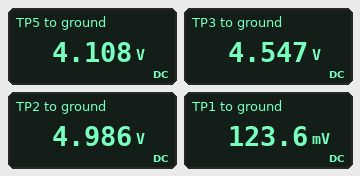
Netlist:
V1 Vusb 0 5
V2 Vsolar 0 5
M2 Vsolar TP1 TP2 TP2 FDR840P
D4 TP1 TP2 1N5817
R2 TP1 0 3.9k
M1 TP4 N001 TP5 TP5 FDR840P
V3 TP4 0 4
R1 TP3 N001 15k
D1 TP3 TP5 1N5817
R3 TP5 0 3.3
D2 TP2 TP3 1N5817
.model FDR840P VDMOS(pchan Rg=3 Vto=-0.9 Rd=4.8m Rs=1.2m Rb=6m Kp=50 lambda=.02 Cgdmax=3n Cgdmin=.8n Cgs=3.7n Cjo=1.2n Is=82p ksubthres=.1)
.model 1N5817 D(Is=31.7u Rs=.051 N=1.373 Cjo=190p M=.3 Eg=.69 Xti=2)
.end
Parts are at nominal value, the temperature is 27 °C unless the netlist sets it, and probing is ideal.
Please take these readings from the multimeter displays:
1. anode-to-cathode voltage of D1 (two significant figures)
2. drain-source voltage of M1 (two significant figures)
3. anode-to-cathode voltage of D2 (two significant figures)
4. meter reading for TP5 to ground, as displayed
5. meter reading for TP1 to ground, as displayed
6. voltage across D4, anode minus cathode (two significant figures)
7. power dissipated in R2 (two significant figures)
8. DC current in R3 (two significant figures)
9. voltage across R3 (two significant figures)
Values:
440 mV
-110 mV
440 mV
4.108 V
123.6 mV
-4.9 V
3.9 µW
1.2 A
4.1 V
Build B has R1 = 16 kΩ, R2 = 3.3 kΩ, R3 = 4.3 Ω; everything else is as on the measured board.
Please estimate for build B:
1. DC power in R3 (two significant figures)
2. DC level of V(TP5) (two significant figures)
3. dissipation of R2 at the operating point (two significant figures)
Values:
4.0 W
4.2 V
3.3 µW
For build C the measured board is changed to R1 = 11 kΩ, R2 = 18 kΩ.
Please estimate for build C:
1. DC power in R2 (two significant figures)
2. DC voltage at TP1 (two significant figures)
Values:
18 µW
570 mV
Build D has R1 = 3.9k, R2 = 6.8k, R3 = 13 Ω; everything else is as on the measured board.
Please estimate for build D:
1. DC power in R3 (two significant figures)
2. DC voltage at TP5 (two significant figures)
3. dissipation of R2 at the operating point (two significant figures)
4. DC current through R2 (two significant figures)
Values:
1.4 W
4.3 V
6.8 µW
32 µA
